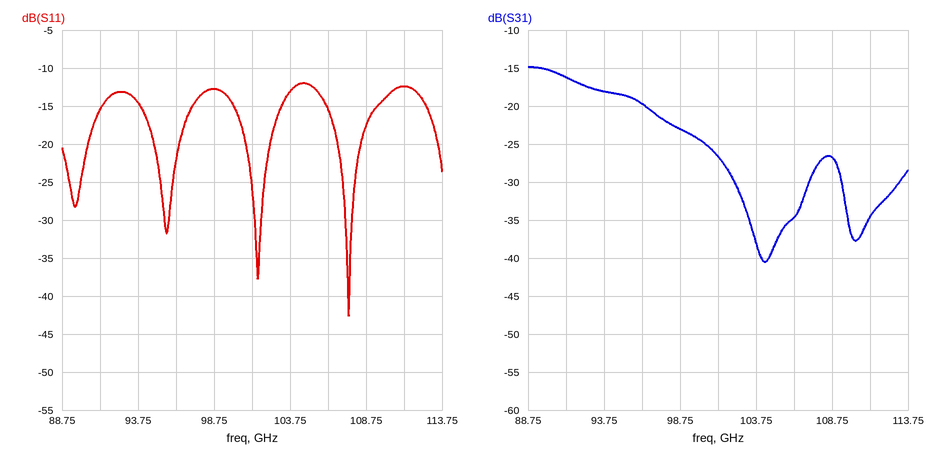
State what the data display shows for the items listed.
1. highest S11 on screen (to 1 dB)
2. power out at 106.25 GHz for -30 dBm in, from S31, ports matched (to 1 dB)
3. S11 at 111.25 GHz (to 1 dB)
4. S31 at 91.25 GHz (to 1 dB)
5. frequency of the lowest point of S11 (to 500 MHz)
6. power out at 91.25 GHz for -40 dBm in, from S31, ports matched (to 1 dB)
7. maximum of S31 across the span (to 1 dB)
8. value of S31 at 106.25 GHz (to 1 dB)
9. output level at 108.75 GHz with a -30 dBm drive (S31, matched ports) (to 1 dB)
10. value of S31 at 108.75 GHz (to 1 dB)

-12 dB
-65 dBm
-12 dB
-16 dB
107.5 GHz
-56 dBm
-15 dB
-35 dB
-57 dBm
-27 dB
